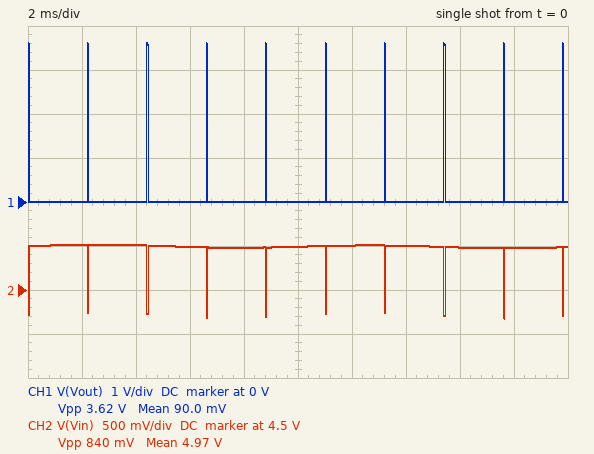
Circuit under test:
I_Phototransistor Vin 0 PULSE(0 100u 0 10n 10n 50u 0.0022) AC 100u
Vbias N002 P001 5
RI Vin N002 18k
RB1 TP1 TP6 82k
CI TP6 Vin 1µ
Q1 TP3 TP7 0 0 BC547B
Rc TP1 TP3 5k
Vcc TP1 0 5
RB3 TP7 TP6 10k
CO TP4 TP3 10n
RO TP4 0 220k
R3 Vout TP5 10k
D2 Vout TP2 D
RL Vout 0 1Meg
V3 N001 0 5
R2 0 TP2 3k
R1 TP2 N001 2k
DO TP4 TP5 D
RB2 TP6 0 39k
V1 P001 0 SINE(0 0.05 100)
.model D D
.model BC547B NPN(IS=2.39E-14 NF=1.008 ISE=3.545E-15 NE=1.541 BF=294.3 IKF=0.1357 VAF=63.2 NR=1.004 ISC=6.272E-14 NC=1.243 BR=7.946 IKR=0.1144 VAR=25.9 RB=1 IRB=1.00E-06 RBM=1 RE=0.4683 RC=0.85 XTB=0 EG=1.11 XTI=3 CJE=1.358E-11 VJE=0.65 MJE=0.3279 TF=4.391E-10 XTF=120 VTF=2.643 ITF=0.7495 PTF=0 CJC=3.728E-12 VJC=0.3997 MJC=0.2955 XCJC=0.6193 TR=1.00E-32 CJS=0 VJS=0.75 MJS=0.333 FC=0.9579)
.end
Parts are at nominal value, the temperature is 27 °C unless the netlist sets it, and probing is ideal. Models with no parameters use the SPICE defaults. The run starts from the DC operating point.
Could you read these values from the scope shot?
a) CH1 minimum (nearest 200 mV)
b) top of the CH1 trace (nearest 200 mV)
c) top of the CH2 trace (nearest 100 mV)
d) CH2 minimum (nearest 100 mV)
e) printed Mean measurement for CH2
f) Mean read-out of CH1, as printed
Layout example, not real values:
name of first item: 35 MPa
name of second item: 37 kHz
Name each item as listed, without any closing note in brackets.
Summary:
CH1 minimum: 0 V
top of the CH1 trace: 3.6 V
top of the CH2 trace: 5.0 V
CH2 minimum: 4.2 V
printed Mean measurement for CH2: 4.97 V
Mean read-out of CH1, as printed: 90.0 mV
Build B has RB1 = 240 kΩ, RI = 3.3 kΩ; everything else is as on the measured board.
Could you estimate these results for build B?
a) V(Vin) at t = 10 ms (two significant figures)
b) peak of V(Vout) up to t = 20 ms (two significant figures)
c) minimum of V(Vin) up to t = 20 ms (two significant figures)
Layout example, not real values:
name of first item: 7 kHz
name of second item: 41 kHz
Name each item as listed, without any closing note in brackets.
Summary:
V(Vin) at t = 10 ms: 5.0 V
peak of V(Vout) up to t = 20 ms: 3.3 V
minimum of V(Vin) up to t = 20 ms: 4.7 V
